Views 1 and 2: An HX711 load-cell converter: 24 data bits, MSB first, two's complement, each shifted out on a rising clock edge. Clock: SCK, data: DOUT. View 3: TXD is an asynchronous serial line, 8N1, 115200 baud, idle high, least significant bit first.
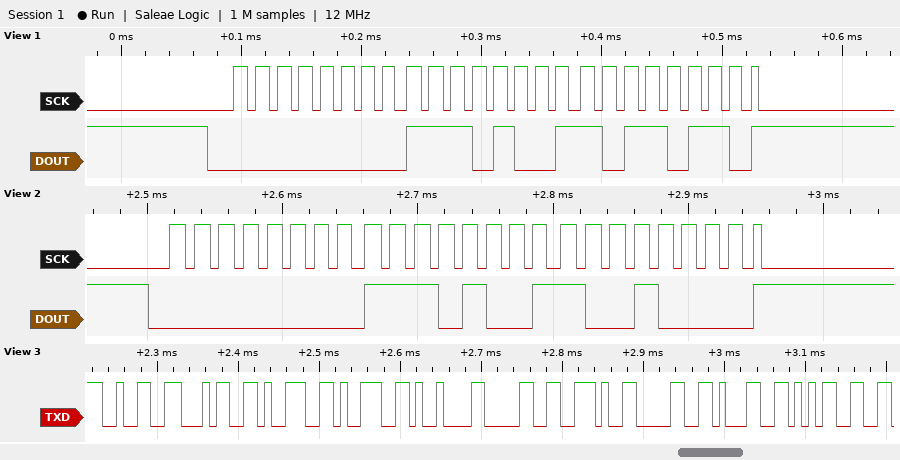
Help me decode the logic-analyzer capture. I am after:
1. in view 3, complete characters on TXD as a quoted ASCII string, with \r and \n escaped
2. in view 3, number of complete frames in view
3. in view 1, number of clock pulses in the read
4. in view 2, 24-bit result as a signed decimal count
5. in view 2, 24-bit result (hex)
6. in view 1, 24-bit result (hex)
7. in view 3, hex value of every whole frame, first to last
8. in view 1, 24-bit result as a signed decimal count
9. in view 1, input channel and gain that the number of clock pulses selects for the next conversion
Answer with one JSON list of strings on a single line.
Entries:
["\"2499\\t0.015\"", "10", "25", "59792", "0x00E990", "0x00E9B6", "32 34 39 39 09 30 2E 30 31 35", "59830", "channel A, gain 128"]
